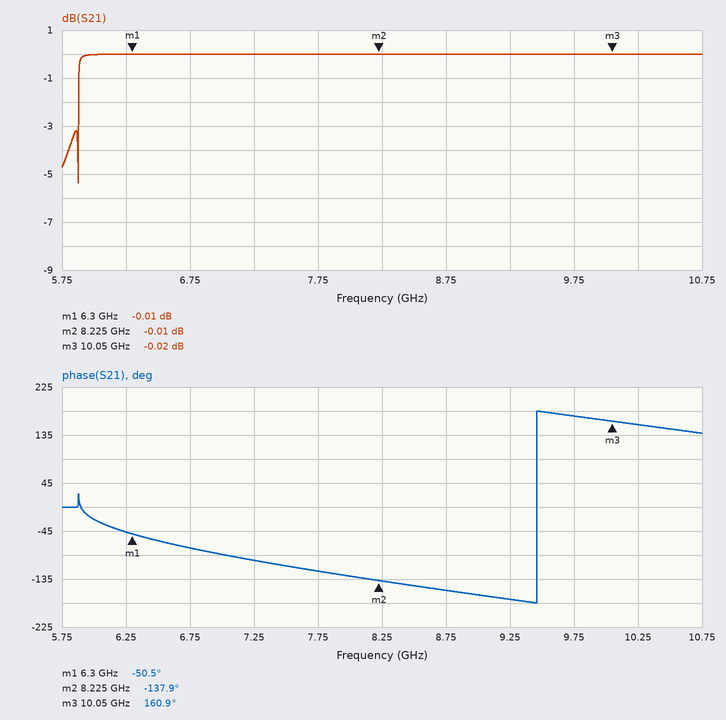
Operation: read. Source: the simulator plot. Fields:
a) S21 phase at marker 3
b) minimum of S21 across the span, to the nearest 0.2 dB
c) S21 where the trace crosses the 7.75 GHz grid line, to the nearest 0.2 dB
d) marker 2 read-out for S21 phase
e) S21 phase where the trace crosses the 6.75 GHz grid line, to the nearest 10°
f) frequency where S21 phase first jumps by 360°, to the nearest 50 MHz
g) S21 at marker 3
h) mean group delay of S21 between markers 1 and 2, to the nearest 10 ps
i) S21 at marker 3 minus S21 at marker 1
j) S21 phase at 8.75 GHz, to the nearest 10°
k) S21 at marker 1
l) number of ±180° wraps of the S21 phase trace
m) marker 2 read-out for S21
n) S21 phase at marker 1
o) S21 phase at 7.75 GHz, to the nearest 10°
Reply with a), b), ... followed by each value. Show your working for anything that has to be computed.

a) 160.9°
b) -5.4 dB
c) 0.0 dB
d) -137.9°
e) -80°
f) 9.45 GHz
g) -0.02 dB
h) −(-137.9° − (-50.5°))/(360° × 1.925 GHz) ≈ 126 ps, so 130 ps to the nearest 10 ps
i) -0.02 − (-0.01) = -0.01 dB
j) -160°
k) -0.01 dB
l) 1
m) -0.01 dB
n) -50.5°
o) -120°
